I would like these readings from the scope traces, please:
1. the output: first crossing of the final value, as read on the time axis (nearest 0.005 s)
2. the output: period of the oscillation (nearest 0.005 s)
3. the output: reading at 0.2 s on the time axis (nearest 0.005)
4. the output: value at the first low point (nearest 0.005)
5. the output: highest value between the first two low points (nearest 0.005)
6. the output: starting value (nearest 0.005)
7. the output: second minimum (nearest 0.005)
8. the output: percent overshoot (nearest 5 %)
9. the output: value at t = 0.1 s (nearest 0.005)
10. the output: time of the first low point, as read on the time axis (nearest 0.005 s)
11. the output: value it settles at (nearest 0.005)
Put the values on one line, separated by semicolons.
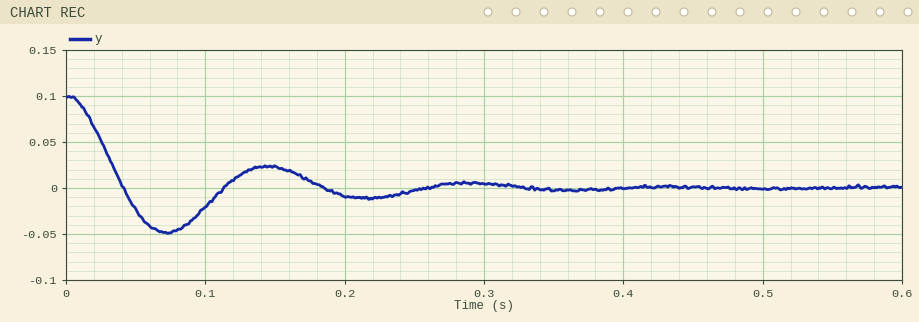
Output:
0.040 s; 0.145 s; -0.010; -0.050; 0.025; 0.100; -0.010; 50 %; -0.020; 0.070 s; 0.000
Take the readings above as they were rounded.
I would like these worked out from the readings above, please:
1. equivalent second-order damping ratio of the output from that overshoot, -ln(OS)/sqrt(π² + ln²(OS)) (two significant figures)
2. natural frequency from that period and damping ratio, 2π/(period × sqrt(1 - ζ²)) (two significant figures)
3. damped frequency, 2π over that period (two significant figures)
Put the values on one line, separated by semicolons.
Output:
0.22; 44 rad/s; 43 rad/s
